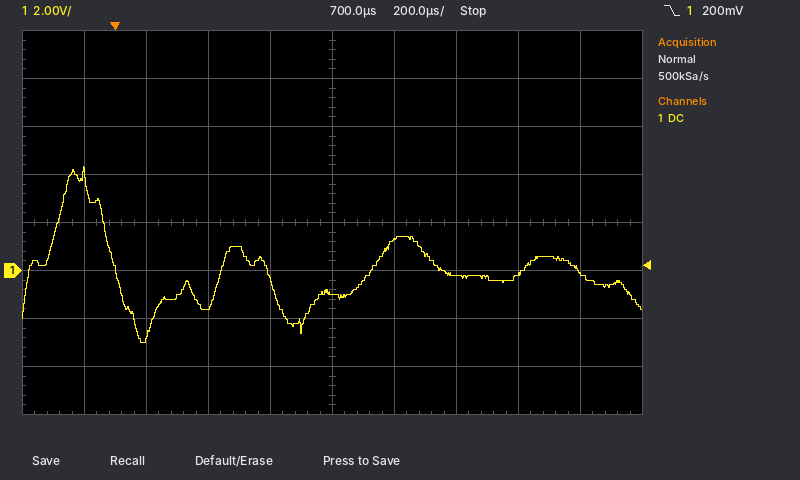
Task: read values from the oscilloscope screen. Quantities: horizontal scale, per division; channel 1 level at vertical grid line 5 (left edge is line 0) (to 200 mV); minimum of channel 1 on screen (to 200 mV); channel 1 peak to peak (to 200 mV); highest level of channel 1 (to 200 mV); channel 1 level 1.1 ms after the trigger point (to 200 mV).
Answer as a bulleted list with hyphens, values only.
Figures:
- 200 µs
- -1.0 V
- -3.0 V
- 7.4 V
- 4.4 V
- -200 mV
